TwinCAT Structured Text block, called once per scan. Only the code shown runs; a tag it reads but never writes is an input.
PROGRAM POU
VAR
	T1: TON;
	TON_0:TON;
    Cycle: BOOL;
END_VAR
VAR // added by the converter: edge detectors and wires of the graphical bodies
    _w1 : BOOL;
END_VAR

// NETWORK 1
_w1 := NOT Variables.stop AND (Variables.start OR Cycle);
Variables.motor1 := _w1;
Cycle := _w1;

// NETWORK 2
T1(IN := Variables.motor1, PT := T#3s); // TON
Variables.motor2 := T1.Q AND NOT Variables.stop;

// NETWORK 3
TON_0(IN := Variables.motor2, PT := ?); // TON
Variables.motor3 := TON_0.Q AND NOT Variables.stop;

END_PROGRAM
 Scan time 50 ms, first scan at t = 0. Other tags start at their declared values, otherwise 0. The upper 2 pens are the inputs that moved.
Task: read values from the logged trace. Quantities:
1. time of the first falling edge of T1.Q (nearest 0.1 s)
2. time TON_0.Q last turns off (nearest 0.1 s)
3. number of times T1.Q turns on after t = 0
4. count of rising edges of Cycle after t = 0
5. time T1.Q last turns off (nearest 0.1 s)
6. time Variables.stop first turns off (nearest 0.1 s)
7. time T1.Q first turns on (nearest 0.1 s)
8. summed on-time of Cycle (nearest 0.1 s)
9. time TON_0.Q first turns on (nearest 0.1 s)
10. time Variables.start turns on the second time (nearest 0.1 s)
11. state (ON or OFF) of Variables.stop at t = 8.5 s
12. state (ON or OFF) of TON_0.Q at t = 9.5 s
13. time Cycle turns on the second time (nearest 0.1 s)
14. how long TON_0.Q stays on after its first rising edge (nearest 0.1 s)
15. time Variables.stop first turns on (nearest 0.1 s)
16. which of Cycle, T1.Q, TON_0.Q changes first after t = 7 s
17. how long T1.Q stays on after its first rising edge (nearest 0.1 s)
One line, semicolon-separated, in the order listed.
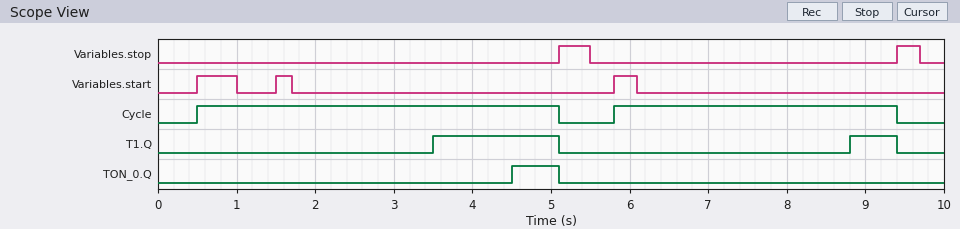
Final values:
5.1 s; 5.1 s; 2; 2; 9.4 s; 5.5 s; 3.5 s; 8.2 s; 4.5 s; 1.5 s; OFF; OFF; 5.8 s; 0.6 s; 5.1 s; T1.Q; 1.6 s
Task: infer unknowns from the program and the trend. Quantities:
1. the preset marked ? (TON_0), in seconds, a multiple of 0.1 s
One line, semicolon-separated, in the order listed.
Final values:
1.0 s
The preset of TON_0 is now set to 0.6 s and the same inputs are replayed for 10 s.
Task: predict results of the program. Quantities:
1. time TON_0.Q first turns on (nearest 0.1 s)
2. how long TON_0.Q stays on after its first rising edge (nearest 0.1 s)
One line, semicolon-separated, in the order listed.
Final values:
4.1 s; 1.0 s
